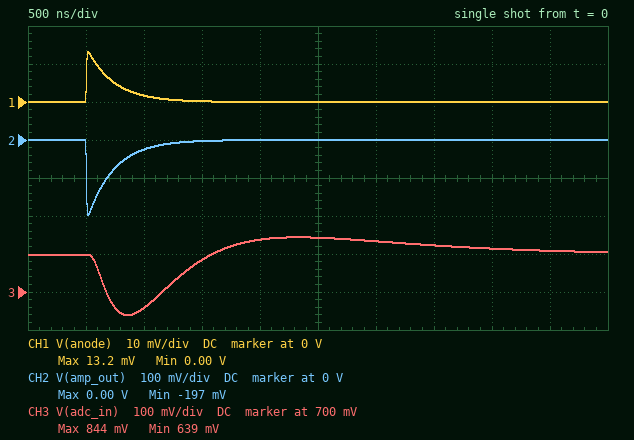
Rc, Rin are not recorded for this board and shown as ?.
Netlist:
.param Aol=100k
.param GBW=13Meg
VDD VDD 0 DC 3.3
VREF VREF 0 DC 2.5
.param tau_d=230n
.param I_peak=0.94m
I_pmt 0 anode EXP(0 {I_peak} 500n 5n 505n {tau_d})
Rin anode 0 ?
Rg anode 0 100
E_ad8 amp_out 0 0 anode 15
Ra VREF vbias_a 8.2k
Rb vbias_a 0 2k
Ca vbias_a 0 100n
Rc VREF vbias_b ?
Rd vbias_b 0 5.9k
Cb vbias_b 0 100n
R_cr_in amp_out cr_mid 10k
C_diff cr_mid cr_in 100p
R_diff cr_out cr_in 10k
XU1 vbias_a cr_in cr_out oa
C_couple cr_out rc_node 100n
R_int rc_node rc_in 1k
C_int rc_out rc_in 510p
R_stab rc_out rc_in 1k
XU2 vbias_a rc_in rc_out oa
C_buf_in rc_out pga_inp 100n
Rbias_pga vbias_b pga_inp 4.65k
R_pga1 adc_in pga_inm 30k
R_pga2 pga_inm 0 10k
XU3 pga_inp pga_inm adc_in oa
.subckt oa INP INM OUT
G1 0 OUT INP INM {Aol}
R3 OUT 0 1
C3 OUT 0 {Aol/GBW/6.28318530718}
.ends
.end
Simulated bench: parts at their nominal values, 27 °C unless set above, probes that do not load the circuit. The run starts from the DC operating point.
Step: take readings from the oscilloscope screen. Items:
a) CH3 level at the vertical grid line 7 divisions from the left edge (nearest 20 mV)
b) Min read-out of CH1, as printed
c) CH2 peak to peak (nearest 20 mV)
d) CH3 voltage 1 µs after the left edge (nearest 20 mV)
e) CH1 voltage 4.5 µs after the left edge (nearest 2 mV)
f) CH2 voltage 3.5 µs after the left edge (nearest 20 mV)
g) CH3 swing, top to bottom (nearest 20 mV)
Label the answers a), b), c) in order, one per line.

a) 820 mV
b) 0.00 V
c) 200 mV
d) 660 mV
e) 0 V
f) 0 V
g) 200 mV
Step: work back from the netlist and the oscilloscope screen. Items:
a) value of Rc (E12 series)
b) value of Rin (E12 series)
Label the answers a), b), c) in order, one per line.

a) 68 kΩ
b) 18 Ω
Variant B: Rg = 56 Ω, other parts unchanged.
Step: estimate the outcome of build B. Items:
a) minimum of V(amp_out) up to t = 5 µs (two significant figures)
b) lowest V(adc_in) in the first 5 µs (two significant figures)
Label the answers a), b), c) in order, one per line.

a) -180 mV
b) 660 mV
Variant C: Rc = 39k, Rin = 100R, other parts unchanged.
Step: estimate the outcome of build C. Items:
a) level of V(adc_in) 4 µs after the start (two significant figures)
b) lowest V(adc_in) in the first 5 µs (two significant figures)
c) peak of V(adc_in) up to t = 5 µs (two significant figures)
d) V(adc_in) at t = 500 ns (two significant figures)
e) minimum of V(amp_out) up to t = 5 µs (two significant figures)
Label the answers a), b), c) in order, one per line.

a) 1.4 V
b) 790 mV
c) 1.5 V
d) 1.3 V
e) -650 mV
